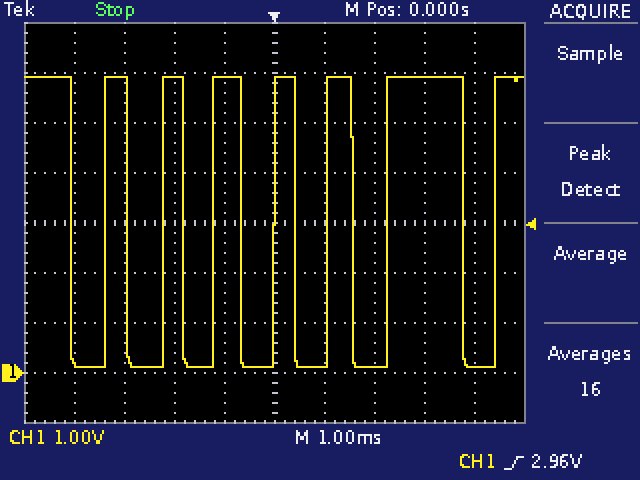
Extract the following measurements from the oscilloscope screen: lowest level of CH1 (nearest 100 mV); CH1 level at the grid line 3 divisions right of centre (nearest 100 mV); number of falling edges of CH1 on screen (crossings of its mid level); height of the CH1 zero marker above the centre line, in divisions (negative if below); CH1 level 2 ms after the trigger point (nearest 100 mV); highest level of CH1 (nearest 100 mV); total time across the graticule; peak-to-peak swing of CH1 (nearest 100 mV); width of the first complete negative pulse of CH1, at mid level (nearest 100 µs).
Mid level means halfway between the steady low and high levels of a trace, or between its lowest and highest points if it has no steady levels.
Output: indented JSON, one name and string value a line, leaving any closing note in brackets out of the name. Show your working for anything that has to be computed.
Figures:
{
  "lowest level of CH1": "100 mV",
  "CH1 level at the grid line 3 divisions right of centre": "5.9 V",
  "number of falling edges of CH1 on screen": "7",
  "height of the CH1 zero marker above the centre line, in divisions": "-3.0 div",
  "CH1 level 2 ms after the trigger point": "100 mV",
  "highest level of CH1": "5.9 V",
  "total time across the graticule": "10 ms",
  "peak-to-peak swing of CH1": "5.9 V − (100 mV) = 5.8 V",
  "width of the first complete negative pulse of CH1, at mid level": "700 µs"
}
